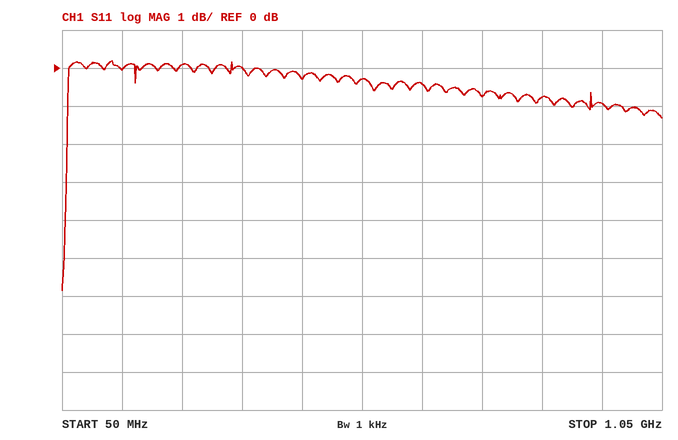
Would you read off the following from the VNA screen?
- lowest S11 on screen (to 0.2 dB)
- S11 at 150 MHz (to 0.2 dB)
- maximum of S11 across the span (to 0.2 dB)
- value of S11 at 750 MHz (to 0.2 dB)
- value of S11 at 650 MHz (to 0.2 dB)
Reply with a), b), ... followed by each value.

a) -5.8 dB
b) 0.0 dB
c) 0.2 dB
d) -0.8 dB
e) -0.4 dB
